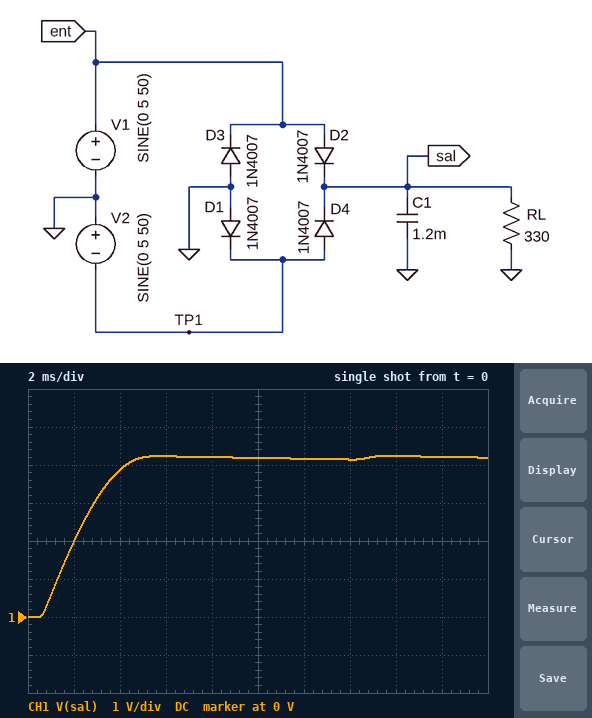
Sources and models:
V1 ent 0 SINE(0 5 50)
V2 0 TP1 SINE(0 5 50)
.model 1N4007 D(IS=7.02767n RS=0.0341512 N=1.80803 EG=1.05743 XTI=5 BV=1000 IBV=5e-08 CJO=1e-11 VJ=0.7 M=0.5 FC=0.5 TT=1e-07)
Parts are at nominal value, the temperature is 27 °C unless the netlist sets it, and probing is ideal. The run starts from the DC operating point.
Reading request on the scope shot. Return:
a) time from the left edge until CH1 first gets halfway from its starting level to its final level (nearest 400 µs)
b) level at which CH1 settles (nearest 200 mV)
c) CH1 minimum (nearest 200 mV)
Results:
2.0 ms
4.2 V
0 V
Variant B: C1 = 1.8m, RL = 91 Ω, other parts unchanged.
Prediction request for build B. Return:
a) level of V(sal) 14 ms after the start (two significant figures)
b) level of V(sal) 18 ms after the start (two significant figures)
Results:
4.0 V
4.1 V
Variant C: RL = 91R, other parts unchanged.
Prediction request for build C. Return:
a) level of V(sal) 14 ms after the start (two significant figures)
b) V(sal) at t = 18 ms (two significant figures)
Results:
3.9 V
4.1 V
